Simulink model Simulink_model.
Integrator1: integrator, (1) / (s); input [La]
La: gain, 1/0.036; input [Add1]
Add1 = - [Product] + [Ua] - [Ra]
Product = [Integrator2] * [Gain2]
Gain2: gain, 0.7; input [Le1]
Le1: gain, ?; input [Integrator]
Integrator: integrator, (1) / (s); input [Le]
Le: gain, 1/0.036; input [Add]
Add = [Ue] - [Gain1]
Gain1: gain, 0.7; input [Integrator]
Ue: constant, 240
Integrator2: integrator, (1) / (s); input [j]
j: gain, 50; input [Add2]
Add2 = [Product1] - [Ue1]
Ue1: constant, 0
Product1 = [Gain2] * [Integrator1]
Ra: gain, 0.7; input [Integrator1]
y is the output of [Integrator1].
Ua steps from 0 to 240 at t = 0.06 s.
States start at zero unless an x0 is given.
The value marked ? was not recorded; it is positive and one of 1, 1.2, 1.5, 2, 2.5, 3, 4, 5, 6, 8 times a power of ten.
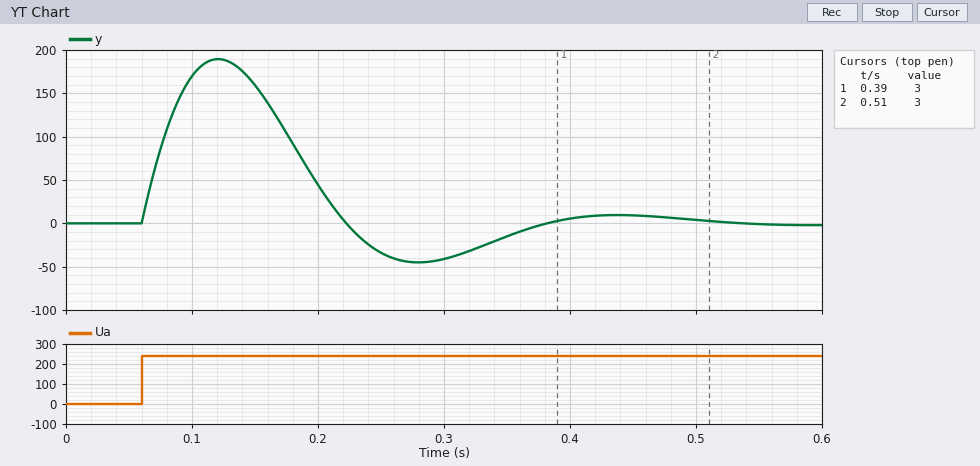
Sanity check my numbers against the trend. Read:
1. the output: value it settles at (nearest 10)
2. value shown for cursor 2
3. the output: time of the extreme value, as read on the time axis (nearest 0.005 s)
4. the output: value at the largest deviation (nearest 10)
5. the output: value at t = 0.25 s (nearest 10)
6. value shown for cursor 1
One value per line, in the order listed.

0
3
0.120 s
190
-30
3
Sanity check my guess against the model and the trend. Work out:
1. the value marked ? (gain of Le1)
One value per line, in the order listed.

0.0025
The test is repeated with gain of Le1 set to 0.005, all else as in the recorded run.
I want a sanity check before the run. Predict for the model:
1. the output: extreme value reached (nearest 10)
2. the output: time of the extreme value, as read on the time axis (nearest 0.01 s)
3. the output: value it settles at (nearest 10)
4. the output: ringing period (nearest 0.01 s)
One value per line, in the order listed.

130
0.10 s
0
0.15 s
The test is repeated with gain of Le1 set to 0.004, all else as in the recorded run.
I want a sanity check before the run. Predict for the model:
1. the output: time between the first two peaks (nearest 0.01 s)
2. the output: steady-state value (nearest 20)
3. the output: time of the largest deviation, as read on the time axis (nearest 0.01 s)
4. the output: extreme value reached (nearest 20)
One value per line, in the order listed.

0.19 s
0
0.10 s
140
